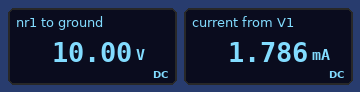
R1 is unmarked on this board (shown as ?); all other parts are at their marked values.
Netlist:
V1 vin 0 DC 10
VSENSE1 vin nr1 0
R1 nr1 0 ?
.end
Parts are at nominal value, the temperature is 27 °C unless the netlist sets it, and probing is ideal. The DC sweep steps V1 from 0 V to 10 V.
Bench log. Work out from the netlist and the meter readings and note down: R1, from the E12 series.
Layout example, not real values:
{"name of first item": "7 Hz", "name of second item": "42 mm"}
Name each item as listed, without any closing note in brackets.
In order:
{"R1, from the E12 series": "5.6 kΩ"}
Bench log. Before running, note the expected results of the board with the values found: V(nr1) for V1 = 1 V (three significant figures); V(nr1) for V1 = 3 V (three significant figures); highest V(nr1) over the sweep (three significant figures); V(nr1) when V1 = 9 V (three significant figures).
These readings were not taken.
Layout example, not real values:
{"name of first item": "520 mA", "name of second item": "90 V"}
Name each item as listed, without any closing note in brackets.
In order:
{"V(nr1) for V1 = 1 V": "1.00 V", "V(nr1) for V1 = 3 V": "3.00 V", "highest V(nr1) over the sweep": "10.0 V", "V(nr1) when V1 = 9 V": "9.00 V"}
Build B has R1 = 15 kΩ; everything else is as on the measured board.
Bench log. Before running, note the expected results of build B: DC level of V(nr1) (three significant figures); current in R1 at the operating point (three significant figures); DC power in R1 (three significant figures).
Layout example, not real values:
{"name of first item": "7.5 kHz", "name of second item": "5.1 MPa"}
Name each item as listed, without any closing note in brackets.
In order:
{"DC level of V(nr1)": "10.0 V", "current in R1 at the operating point": "667 µA", "DC power in R1": "6.67 mW"}
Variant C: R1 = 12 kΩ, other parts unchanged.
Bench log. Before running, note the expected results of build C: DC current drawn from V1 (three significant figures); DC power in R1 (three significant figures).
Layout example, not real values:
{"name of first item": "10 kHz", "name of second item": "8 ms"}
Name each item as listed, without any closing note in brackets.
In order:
{"DC current drawn from V1": "833 µA", "DC power in R1": "8.33 mW"}
